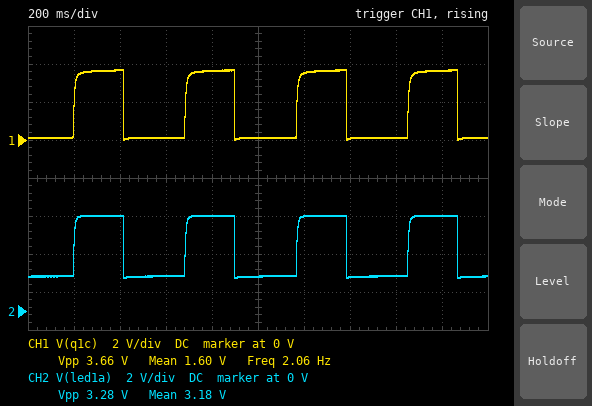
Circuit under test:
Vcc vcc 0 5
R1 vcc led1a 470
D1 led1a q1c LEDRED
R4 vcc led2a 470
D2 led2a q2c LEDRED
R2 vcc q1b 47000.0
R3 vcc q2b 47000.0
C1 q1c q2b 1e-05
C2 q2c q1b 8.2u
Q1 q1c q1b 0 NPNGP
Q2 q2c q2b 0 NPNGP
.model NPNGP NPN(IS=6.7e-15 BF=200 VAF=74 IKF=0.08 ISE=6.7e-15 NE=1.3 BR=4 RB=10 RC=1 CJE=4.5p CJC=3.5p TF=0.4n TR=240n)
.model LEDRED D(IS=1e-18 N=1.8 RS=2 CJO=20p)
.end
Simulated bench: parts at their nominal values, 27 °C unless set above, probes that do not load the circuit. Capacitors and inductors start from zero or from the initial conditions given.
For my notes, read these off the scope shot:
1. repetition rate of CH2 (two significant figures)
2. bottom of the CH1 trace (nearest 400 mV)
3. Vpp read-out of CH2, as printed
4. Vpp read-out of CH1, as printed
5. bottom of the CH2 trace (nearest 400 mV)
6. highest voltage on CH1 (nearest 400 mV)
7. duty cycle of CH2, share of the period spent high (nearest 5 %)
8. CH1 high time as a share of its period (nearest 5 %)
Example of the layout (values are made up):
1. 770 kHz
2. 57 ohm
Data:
1. 2.1 Hz
2. 0 V
3. 3.28 V
4. 3.66 V
5. 1.6 V
6. 3.6 V
7. 45 %
8. 45 %
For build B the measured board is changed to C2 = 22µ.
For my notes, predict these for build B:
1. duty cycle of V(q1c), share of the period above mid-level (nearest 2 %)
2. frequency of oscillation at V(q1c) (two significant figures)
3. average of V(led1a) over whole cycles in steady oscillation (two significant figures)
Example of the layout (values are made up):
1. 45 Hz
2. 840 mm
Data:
1. 68 %
2. 1.2 Hz
3. 4.0 V
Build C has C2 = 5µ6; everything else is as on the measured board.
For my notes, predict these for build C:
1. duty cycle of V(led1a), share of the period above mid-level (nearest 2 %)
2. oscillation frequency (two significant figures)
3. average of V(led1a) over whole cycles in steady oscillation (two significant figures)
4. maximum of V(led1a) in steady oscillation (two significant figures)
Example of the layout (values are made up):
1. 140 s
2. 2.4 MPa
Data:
1. 36 %
2. 2.4 Hz
3. 2.9 V
4. 5.0 V
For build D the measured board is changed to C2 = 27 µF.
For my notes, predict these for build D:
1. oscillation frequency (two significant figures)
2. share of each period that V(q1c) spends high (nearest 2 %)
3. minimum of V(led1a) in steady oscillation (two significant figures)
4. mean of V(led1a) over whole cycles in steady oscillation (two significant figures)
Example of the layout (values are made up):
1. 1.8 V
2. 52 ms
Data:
1. 1.0 Hz
2. 72 %
3. 1.7 V
4. 4.1 V
